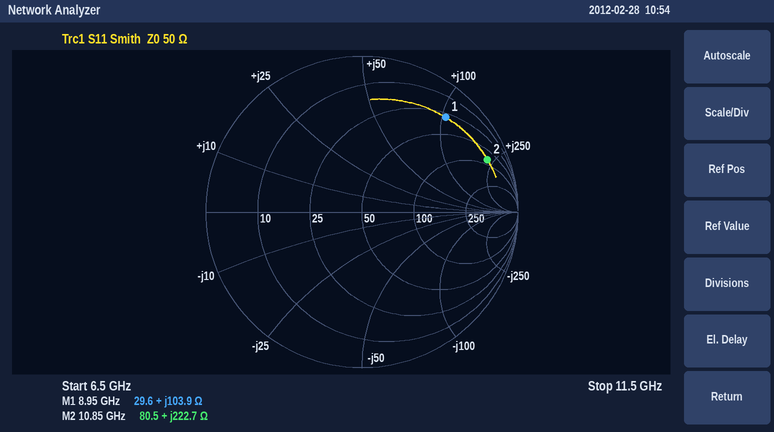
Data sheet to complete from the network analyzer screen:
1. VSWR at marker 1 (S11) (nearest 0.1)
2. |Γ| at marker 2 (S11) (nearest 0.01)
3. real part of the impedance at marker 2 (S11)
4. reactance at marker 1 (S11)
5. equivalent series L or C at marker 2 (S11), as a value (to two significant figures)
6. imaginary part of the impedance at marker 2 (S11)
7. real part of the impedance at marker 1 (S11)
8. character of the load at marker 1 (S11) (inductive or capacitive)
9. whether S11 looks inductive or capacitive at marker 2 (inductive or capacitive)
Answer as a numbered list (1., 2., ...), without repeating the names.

1. 9.5
2. 0.87
3. 80.5 Ω
4. +103.9 Ω
5. 3.3 nH
6. +222.7 Ω
7. 29.6 Ω
8. inductive
9. inductive
